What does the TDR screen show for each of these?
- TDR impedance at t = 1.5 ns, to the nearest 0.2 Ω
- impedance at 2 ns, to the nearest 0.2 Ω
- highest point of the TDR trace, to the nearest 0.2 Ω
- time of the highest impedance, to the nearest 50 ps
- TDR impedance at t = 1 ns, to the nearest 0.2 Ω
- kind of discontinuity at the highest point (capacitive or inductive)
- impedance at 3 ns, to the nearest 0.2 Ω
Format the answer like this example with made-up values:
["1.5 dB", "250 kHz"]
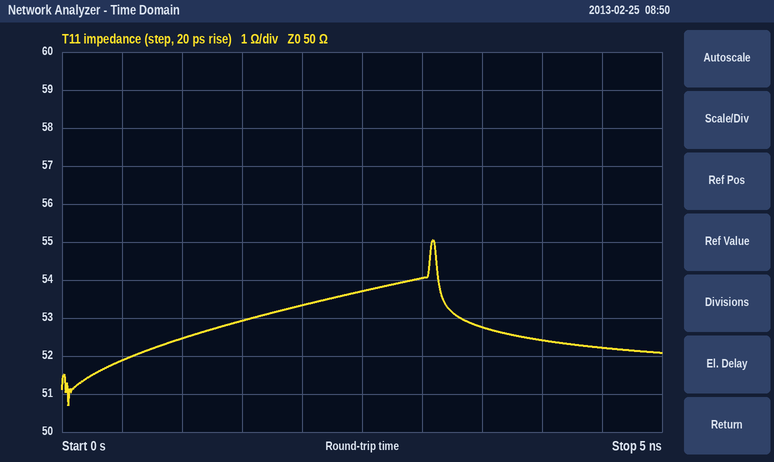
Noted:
["53.0 Ω", "53.4 Ω", "55.0 Ω", "3.10 ns", "52.4 Ω", "inductive", "54.0 Ω"]
